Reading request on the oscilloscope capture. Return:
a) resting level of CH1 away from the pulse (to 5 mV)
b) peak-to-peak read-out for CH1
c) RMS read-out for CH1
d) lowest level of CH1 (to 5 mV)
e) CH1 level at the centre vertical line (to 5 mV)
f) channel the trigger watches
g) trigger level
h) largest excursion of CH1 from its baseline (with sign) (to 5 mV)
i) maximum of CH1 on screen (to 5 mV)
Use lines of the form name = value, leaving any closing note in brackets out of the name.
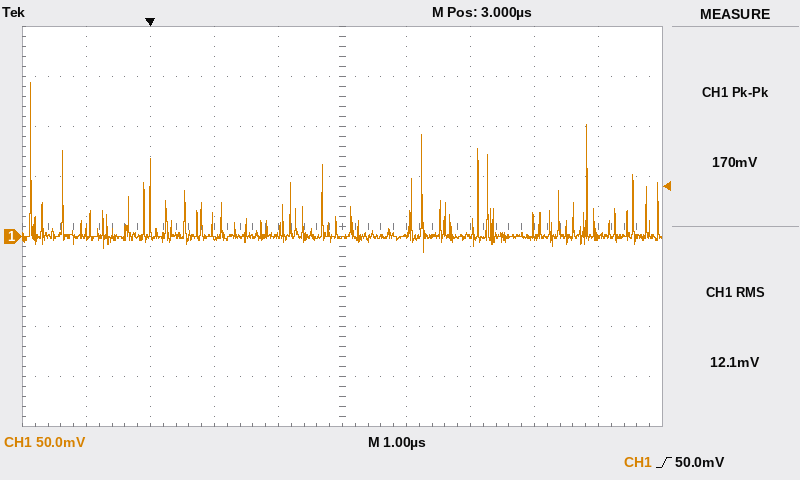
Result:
resting level of CH1 away from the pulse = 0 mV
peak-to-peak read-out for CH1 = 170 mV
RMS read-out for CH1 = 12.1 mV
lowest level of CH1 = -15 mV
CH1 level at the centre vertical line = 0 mV
channel the trigger watches = CH1
trigger level = 50.0 mV
largest excursion of CH1 from its baseline (with sign) = +155 mV
maximum of CH1 on screen = 155 mV
